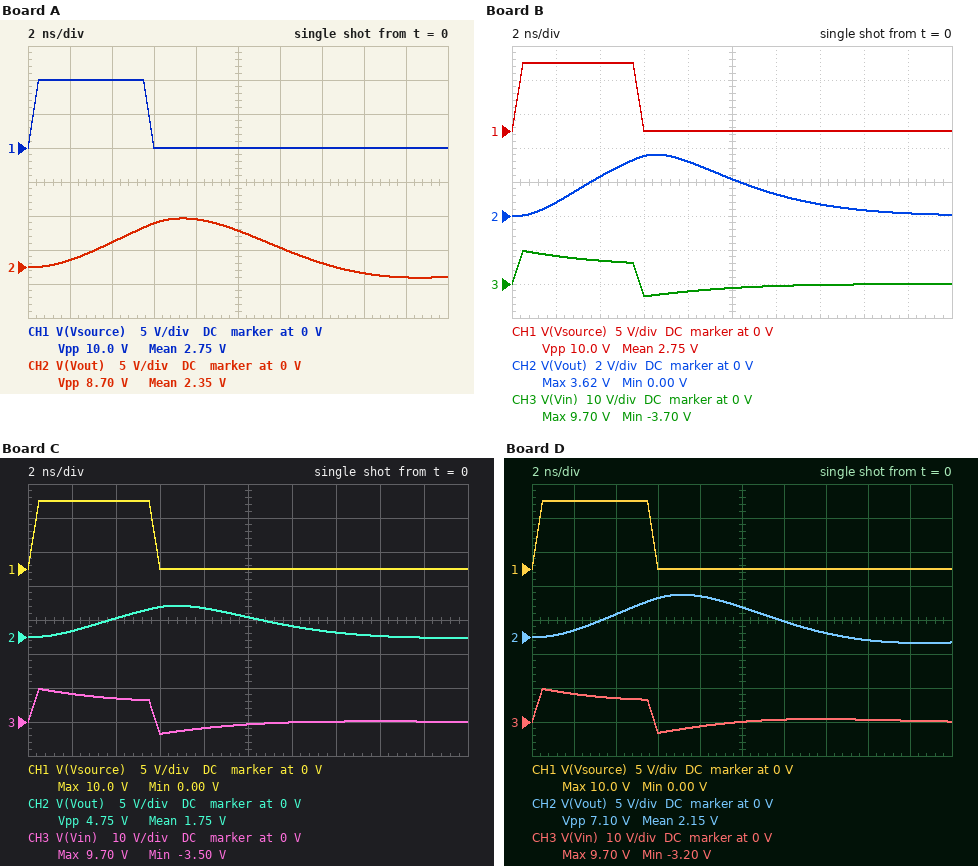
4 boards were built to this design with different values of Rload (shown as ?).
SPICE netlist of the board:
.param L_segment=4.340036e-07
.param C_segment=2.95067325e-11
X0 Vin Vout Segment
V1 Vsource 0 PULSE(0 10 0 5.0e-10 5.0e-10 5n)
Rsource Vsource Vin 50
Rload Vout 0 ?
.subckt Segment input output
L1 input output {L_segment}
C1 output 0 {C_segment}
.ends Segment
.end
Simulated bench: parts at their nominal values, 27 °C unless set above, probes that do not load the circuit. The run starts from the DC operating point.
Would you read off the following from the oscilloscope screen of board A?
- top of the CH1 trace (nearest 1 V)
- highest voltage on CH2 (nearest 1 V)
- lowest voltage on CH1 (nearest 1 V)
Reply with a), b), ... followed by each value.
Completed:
a) 10 V
b) 7 V
c) 0 V
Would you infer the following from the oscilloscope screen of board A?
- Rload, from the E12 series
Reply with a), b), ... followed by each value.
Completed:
a) 220 Ω
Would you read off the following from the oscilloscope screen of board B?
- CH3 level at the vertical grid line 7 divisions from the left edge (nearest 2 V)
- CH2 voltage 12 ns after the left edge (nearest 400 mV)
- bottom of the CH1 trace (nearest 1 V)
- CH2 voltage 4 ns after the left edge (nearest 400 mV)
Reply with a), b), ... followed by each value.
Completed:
a) 0 V
b) 1.2 V
c) 0 V
d) 2.4 V
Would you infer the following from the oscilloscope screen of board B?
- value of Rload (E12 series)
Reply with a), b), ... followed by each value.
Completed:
a) 56 Ω
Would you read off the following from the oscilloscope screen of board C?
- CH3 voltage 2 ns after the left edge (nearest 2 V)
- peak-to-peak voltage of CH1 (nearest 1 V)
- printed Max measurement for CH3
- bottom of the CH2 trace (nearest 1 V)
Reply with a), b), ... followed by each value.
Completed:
a) 8 V
b) 10 V
c) 9.70 V
d) 0 V
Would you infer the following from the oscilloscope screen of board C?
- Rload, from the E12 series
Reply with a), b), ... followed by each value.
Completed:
a) 82 Ω
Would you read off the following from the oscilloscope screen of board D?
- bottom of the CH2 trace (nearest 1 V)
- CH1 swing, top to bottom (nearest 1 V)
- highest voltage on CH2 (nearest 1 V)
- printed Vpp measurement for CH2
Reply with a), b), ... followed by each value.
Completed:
a) -1 V
b) 10 V
c) 6 V
d) 7.10 V
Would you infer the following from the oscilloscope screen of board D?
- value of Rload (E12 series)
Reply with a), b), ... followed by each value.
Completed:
a) 150 Ω
